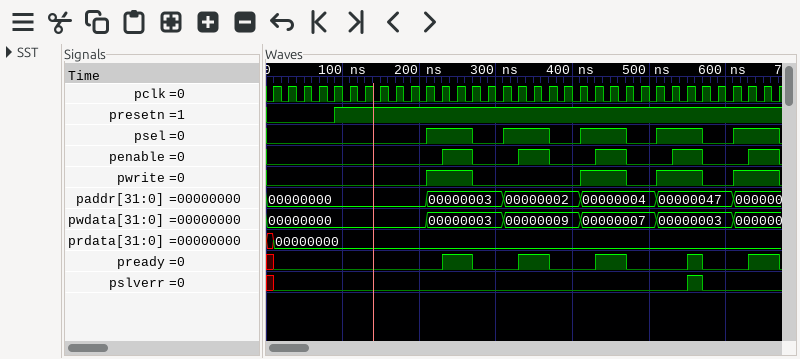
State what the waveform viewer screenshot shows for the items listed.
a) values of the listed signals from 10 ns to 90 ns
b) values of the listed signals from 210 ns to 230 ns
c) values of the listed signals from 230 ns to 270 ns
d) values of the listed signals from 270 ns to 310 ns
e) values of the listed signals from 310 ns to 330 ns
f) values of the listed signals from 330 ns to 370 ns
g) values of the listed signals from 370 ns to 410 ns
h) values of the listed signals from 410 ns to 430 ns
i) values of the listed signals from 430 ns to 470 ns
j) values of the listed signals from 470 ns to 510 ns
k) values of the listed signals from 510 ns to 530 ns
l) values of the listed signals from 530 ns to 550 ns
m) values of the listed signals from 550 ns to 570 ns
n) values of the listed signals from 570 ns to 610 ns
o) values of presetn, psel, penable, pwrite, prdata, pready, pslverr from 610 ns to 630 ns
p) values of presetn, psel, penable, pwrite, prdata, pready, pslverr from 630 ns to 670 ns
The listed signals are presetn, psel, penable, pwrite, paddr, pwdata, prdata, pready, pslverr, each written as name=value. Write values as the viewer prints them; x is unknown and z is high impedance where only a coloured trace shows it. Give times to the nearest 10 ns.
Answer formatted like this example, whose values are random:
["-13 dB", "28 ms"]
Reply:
["presetn=0, psel=0, penable=0, pwrite=0, paddr=00000000, pwdata=00000000, prdata=00000000, pready=0, pslverr=0", "presetn=1, psel=1, penable=0, pwrite=1, paddr=00000003, pwdata=00000003, prdata=00000000, pready=0, pslverr=0", "presetn=1, psel=1, penable=1, pwrite=1, paddr=00000003, pwdata=00000003, prdata=00000000, pready=1, pslverr=0", "presetn=1, psel=0, penable=0, pwrite=0, paddr=00000003, pwdata=00000003, prdata=00000000, pready=0, pslverr=0", "presetn=1, psel=1, penable=0, pwrite=0, paddr=00000002, pwdata=00000009, prdata=00000000, pready=0, pslverr=0", "presetn=1, psel=1, penable=1, pwrite=0, paddr=00000002, pwdata=00000009, prdata=00000000, pready=1, pslverr=0", "presetn=1, psel=0, penable=0, pwrite=0, paddr=00000002, pwdata=00000009, prdata=00000000, pready=0, pslverr=0", "presetn=1, psel=1, penable=0, pwrite=1, paddr=00000004, pwdata=00000007, prdata=00000000, pready=0, pslverr=0", "presetn=1, psel=1, penable=1, pwrite=1, paddr=00000004, pwdata=00000007, prdata=00000000, pready=1, pslverr=0", "presetn=1, psel=0, penable=0, pwrite=0, paddr=00000004, pwdata=00000007, prdata=00000000, pready=0, pslverr=0", "presetn=1, psel=1, penable=0, pwrite=1, paddr=00000047, pwdata=00000003, prdata=00000000, pready=0, pslverr=0", "presetn=1, psel=1, penable=1, pwrite=1, paddr=00000047, pwdata=00000003, prdata=00000000, pready=0, pslverr=0", "presetn=1, psel=1, penable=1, pwrite=1, paddr=00000047, pwdata=00000003, prdata=00000000, pready=1, pslverr=1", "presetn=1, psel=0, penable=0, pwrite=0, paddr=00000047, pwdata=00000003, prdata=00000000, pready=0, pslverr=0", "presetn=1, psel=1, penable=0, pwrite=1, prdata=00000000, pready=0, pslverr=0", "presetn=1, psel=1, penable=1, pwrite=1, prdata=00000000, pready=1, pslverr=0"]
